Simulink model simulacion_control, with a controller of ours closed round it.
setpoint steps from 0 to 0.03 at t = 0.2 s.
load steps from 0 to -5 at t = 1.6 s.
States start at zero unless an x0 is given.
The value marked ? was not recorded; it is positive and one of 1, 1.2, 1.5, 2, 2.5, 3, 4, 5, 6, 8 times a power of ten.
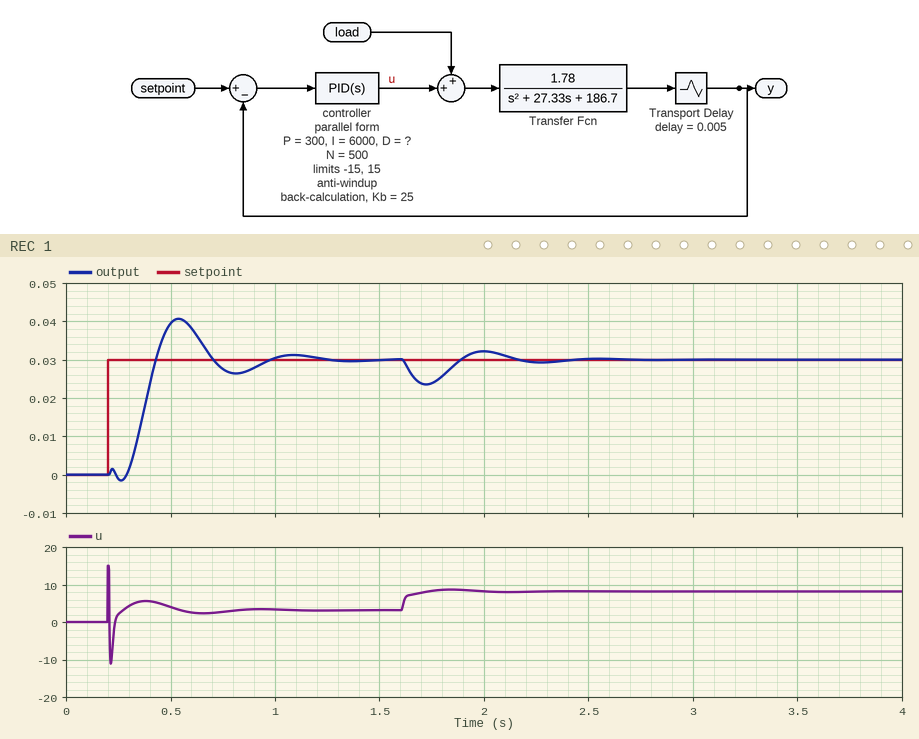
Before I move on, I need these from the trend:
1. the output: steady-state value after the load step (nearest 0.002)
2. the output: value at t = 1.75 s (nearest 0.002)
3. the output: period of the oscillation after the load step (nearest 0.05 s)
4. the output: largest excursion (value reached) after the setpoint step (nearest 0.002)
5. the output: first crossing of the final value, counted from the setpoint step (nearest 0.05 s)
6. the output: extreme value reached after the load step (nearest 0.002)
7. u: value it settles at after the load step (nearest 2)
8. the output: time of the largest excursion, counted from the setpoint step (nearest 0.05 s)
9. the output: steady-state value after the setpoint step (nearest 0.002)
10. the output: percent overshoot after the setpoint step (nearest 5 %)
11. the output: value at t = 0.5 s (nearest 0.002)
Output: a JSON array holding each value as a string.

["0.030", "0.024", "0.55 s", "0.040", "0.25 s", "0.024", "8", "0.35 s", "0.030", "35 %", "0.040"]
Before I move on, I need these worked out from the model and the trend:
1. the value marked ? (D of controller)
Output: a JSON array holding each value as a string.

["30"]
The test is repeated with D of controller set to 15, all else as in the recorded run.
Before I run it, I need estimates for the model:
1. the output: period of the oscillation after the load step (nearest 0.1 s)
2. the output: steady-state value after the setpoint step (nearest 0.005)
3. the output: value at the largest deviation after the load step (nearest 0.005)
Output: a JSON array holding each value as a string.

["0.4 s", "0.030", "0.020"]
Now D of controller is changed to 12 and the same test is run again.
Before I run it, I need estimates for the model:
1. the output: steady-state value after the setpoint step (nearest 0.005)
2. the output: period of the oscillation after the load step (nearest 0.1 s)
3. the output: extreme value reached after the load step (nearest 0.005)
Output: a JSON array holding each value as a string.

["0.030", "0.4 s", "0.020"]
